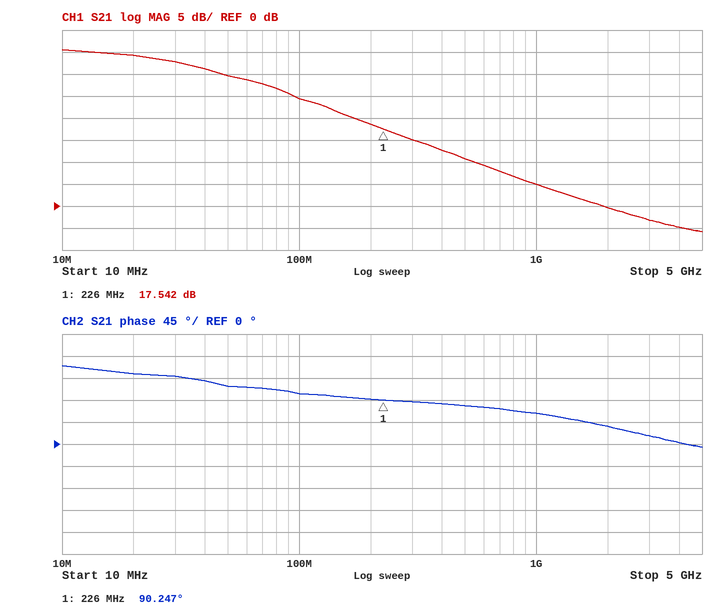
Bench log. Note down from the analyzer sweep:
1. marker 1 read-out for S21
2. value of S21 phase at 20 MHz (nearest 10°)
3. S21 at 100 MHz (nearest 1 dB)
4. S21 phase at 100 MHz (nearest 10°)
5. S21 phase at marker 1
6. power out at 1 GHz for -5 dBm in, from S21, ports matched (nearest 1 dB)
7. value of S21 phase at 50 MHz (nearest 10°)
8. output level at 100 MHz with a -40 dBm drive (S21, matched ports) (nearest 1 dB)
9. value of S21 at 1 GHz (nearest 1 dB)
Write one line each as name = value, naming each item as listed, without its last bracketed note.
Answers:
marker 1 read-out for S21 = 17.542 dB
value of S21 phase at 20 MHz = 140°
S21 at 100 MHz = 24 dB
S21 phase at 100 MHz = 100°
S21 phase at marker 1 = 90.247°
power out at 1 GHz for -5 dBm in, from S21, ports matched = 0 dBm
value of S21 phase at 50 MHz = 120°
output level at 100 MHz with a -40 dBm drive (S21, matched ports) = -16 dBm
value of S21 at 1 GHz = 5 dB
